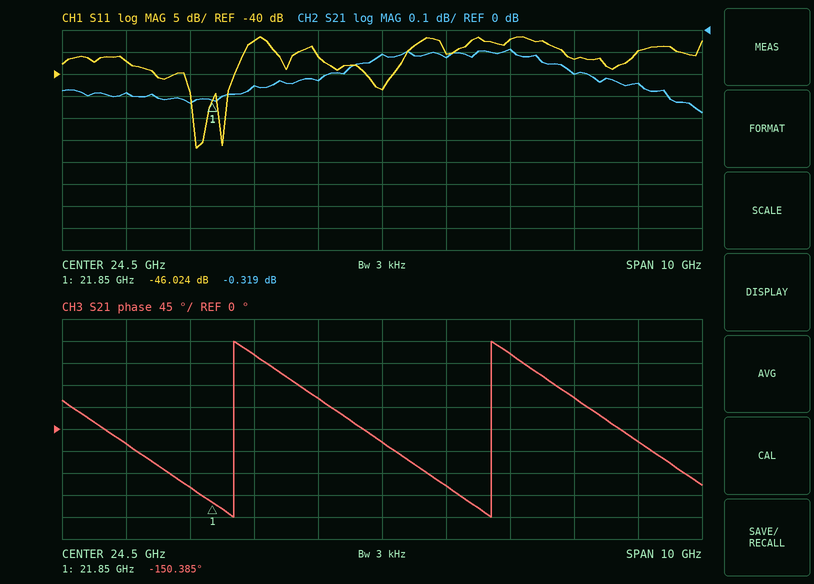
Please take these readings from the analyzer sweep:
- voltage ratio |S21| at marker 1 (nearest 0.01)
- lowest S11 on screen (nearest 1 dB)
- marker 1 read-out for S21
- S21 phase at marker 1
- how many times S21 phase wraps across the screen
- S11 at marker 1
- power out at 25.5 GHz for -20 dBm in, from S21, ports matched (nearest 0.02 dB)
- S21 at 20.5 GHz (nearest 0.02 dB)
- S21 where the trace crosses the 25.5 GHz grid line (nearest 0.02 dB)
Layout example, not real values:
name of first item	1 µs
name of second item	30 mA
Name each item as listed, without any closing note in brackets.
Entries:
voltage ratio |S21| at marker 1	0.96
lowest S11 on screen	-57 dB
marker 1 read-out for S21	-0.319 dB
S21 phase at marker 1	-150.385°
how many times S21 phase wraps across the screen	2
S11 at marker 1	-46.024 dB
power out at 25.5 GHz for -20 dBm in, from S21, ports matched	-20.12 dBm
S21 at 20.5 GHz	-0.28 dB
S21 where the trace crosses the 25.5 GHz grid line	-0.12 dB
